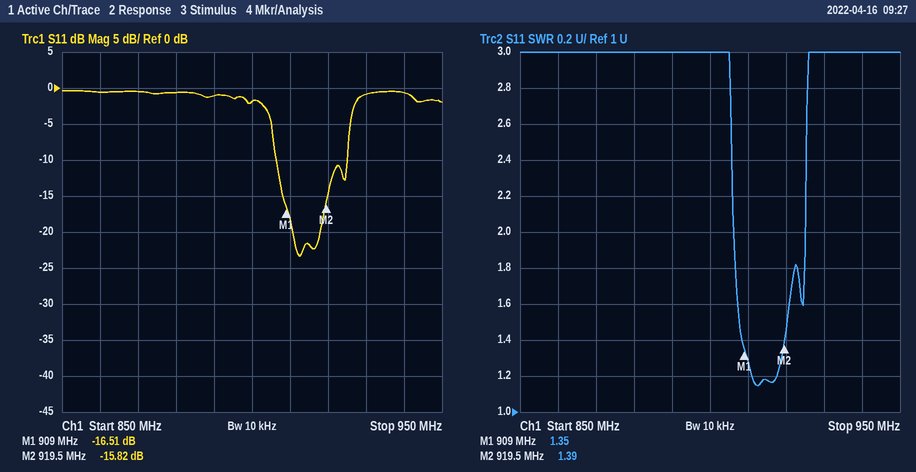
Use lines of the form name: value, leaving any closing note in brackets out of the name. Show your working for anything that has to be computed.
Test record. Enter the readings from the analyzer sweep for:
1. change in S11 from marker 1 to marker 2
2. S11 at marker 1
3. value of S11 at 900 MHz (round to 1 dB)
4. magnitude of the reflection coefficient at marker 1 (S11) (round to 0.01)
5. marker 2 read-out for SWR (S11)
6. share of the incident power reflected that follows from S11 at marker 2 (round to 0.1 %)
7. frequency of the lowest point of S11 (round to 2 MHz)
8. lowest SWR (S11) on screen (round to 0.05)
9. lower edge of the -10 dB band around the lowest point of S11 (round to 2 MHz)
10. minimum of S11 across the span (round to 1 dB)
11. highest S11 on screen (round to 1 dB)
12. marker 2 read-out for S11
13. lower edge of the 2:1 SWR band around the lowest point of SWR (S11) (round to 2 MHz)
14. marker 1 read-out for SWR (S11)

change in S11 from marker 1 to marker 2: -15.82 − (-16.51) = 0.69 dB
S11 at marker 1: -16.51 dB
value of S11 at 900 MHz: -2 dB
magnitude of the reflection coefficient at marker 1 (S11): 10^(-16.51/20) ≈ 0.15
marker 2 read-out for SWR: 1.39
share of the incident power reflected that follows from S11 at marker 2: 10^(-15.82/10) ≈ 2.6 %
frequency of the lowest point of S11: 912 MHz
lowest SWR (S11) on screen: 1.15
lower edge of the -10 dB band around the lowest point of S11: 906 MHz
minimum of S11 across the span: -23 dB
highest S11 on screen: 0 dB
marker 2 read-out for S11: -15.82 dB
lower edge of the 2:1 SWR band around the lowest point of SWR (S11): 906 MHz
marker 1 read-out for SWR: 1.35
